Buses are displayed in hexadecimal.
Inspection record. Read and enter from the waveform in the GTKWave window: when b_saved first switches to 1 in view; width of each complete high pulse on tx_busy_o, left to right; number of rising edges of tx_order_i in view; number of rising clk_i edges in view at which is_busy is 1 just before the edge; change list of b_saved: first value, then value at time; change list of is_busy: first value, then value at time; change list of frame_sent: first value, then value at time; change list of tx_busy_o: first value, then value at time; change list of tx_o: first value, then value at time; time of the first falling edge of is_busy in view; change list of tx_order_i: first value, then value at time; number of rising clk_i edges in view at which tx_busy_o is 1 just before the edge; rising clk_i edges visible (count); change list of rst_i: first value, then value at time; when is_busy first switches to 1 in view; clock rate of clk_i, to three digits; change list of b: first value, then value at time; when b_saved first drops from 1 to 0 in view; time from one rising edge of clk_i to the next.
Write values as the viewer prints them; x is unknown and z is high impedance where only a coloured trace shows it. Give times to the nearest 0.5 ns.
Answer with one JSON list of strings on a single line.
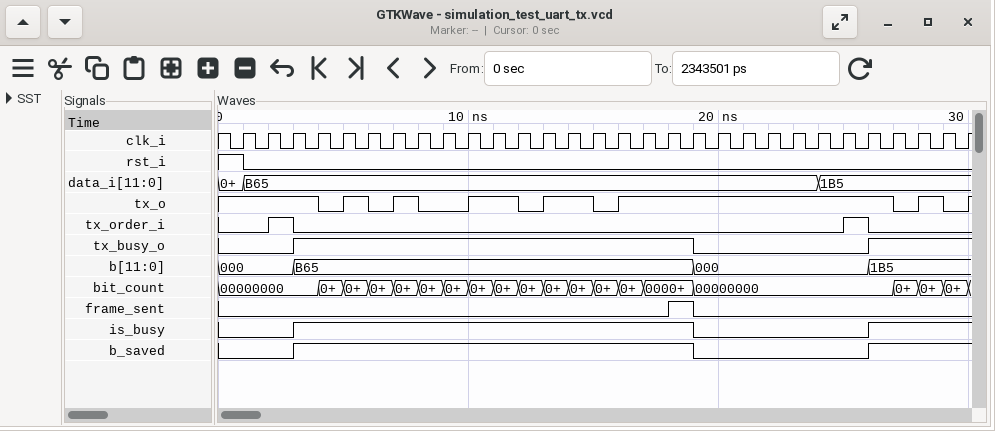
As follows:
["3 ns", "16 ns", "2", "20", "0, 1 at 3 ns, 0 at 19 ns, 1 at 26 ns", "0, 1 at 3 ns, 0 at 19 ns, 1 at 26 ns", "0, 1 at 18 ns, 0 at 19 ns", "0, 1 at 3 ns, 0 at 19 ns, 1 at 26 ns", "1, 0 at 4 ns, 1 at 5 ns, 0 at 6 ns, 1 at 7 ns, 0 at 8 ns, 1 at 10 ns, 0 at 12 ns, 1 at 13 ns, 0 at 15 ns, 1 at 16 ns, 0 at 27 ns, 1 at 28 ns, 0 at 29 ns, 1 at 30 ns", "19 ns", "0, 1 at 2 ns, 0 at 3 ns, 1 at 25 ns, 0 at 26 ns", "20", "30", "1, 0 at 1 ns", "3 ns", "1.00 GHz", "000, B65 at 3 ns, 000 at 19 ns, 1B5 at 26 ns", "19 ns", "1 ns"]
